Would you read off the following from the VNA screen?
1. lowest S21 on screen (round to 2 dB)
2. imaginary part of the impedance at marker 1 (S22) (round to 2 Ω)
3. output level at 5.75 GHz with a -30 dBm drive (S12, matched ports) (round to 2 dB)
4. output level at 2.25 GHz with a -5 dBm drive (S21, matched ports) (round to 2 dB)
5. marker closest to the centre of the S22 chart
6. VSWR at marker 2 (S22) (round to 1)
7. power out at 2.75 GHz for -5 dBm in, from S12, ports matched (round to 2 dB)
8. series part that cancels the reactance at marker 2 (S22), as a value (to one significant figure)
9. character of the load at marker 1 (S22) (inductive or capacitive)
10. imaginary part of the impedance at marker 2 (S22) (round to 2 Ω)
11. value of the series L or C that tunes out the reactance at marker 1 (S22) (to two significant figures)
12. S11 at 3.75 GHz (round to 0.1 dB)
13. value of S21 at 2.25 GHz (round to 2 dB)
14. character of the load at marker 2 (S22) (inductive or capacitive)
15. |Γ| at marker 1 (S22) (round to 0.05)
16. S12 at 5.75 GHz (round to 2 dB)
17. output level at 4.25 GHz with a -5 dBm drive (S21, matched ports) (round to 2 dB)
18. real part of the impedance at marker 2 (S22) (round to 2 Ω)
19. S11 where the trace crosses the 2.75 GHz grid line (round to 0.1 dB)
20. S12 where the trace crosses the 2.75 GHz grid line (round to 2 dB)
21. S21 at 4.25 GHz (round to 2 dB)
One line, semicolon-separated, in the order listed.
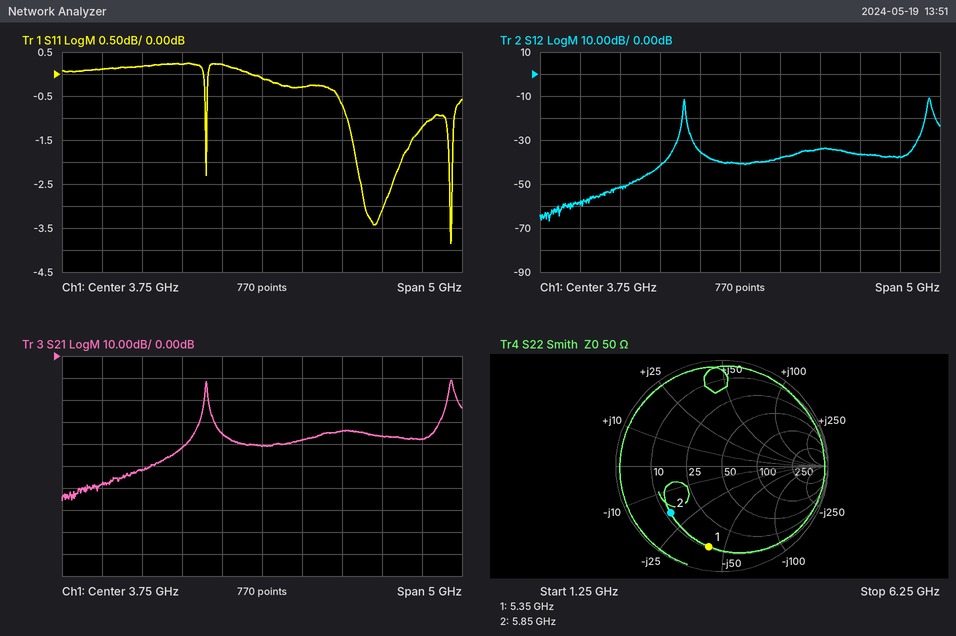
-66 dB; -42 Ω; -68 dBm; -56 dBm; marker 2; 5; -46 dBm; 500 pH; capacitive; -18 Ω; 1.2 nH; -0.1 dB; -52 dB; capacitive; 0.75; -38 dB; -44 dBm; 12 Ω; 0.2 dB; -42 dB; -38 dB
